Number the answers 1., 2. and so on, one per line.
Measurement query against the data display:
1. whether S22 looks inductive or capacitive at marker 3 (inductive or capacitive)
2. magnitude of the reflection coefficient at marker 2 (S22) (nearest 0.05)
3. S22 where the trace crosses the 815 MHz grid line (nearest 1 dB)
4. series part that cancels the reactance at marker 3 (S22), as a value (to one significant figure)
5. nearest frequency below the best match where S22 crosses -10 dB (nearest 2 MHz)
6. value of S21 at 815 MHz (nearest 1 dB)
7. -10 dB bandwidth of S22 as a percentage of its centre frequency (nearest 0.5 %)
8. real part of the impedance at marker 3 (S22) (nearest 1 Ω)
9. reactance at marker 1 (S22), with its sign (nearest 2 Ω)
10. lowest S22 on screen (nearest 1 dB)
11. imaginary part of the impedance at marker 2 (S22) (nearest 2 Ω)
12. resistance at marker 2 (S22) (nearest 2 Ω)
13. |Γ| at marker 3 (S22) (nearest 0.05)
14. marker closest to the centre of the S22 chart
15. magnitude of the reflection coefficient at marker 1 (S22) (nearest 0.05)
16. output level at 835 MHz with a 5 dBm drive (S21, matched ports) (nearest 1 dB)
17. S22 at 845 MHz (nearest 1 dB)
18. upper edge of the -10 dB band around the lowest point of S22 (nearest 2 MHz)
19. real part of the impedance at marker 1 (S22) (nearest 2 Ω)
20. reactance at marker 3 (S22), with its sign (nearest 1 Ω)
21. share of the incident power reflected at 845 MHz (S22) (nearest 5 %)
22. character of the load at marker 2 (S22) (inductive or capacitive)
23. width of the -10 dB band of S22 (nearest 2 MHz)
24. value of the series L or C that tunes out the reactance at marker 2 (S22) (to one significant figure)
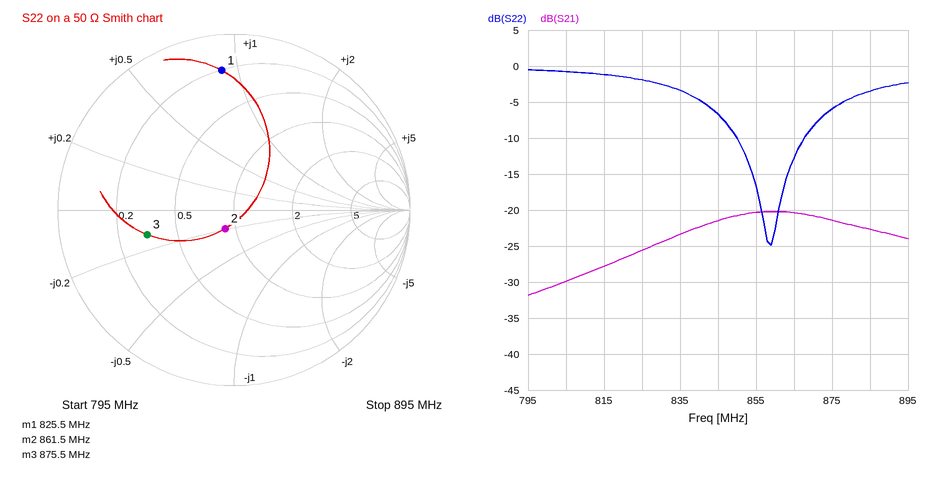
1. capacitive
2. 0.10
3. -1 dB
4. 1 nH
5. 850 MHz
6. -28 dB
7. 2.0 %
8. 16 Ω
9. +44 Ω
10. -25 dB
11. -10 Ω
12. 44 Ω
13. 0.50
14. marker 2
15. 0.80
16. -18 dBm
17. -7 dB
18. 868 MHz
19. 10 Ω
20. -6 Ω
21. 20 %
22. capacitive
23. 18 MHz
24. 2 nH
